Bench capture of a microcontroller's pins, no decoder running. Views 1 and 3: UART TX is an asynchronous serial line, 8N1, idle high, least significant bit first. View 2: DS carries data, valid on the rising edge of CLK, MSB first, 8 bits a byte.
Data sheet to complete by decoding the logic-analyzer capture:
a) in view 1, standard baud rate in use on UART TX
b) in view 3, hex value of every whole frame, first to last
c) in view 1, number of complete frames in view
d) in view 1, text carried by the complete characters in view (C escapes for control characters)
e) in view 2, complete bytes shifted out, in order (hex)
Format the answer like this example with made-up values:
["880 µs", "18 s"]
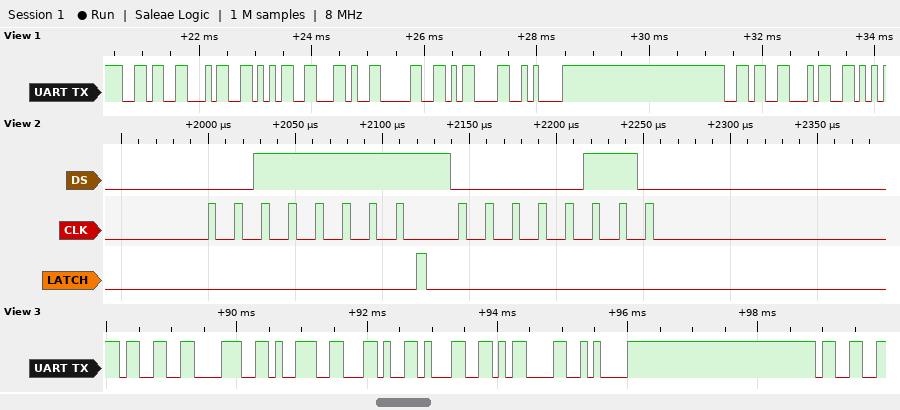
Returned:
["9600 baud", "33 38 39 2C 31 0D 0A 33", "9", "\"645,0\\r\\n64\"", "3F 06"]
